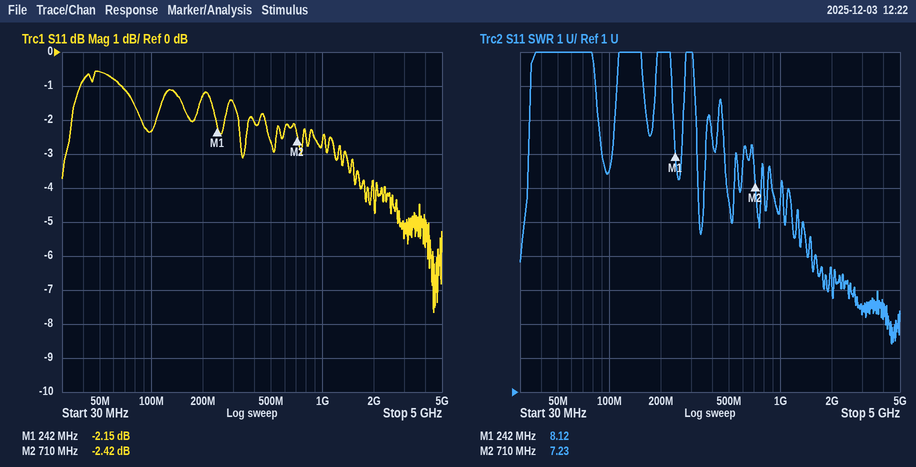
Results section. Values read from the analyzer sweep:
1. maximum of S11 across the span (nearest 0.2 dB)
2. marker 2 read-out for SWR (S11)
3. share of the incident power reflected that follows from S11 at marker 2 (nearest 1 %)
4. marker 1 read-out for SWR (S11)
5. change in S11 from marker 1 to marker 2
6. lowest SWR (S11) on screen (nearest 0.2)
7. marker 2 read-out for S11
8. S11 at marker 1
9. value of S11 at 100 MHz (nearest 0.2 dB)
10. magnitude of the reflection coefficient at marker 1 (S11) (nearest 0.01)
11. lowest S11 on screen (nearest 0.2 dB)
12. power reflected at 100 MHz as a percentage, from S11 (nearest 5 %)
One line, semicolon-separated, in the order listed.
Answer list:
-0.6 dB; 7.23; 57 %; 8.12; -0.27 dB; 2.4; -2.42 dB; -2.15 dB; -2.4 dB; 0.78; -7.6 dB; 60 %
